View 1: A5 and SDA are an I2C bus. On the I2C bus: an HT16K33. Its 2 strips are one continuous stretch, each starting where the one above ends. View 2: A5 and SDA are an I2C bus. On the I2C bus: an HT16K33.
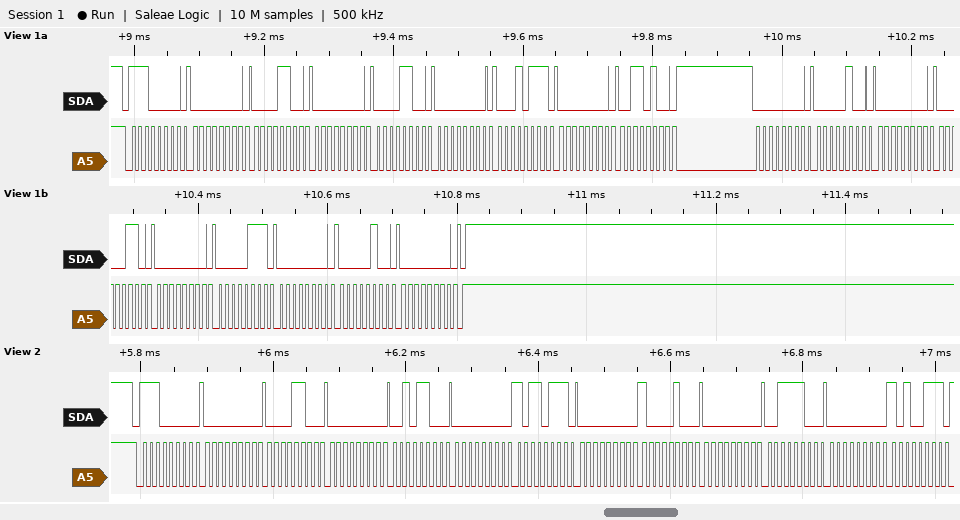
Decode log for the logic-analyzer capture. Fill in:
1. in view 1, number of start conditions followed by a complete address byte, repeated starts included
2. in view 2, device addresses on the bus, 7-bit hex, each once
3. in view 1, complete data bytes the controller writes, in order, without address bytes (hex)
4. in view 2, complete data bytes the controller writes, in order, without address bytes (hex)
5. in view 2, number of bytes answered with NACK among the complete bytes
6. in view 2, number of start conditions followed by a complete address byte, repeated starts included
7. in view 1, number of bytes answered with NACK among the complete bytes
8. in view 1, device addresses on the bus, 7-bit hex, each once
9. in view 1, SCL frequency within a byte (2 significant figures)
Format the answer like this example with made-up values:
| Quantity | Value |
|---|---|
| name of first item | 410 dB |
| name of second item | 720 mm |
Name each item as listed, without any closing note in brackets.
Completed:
| Quantity | Value |
|---|---|
| in view 1, number of start conditions followed by a complete address byte, repeated starts included | 1 |
| in view 2, device addresses on the bus, 7-bit hex, each once | 0x70 |
| in view 1, complete data bytes the controller writes, in order, without address bytes | 00 0C 00 0C 00 17 00 34 00 04 00 06 00 07 00 04 00 |
| in view 2, complete data bytes the controller writes, in order, without address bytes | 00 0C 00 2C 00 B7 00 84 00 3C 00 A7 |
| in view 2, number of bytes answered with NACK among the complete bytes | 0 |
| in view 2, number of start conditions followed by a complete address byte, repeated starts included | 1 |
| in view 1, number of bytes answered with NACK among the complete bytes | 0 |
| in view 1, device addresses on the bus, 7-bit hex, each once | 0x70 |
| in view 1, SCL frequency within a byte | 100 kHz |
